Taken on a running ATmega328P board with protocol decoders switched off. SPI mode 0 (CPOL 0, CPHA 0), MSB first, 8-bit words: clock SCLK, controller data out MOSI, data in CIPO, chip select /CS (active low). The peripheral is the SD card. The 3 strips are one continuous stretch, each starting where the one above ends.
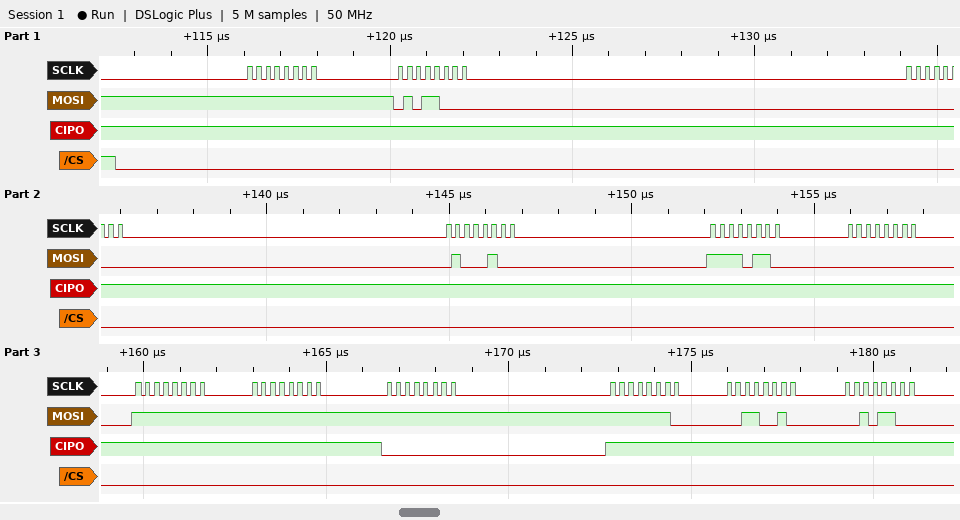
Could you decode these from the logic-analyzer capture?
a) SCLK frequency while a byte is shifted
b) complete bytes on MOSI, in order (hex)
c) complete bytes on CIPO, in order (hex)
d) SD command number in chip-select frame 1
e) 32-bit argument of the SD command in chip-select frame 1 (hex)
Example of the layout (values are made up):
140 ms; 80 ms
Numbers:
4 MHz; FF 58 00 44 F6 00 FF FF FF FE 32 2C; FF FF FF FF FF FF FF FF 00 FF FF FF; CMD24; 0x0044F600
